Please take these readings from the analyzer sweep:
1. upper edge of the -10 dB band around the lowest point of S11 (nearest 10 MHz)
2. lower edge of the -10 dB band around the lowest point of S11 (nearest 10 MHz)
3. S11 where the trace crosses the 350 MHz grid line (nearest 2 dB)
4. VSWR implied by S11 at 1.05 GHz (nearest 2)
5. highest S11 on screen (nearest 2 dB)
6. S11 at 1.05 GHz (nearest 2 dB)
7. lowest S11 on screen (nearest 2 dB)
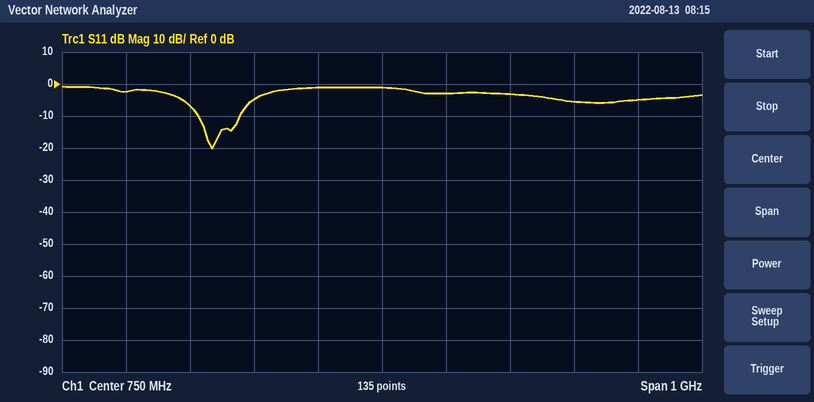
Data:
530 MHz
460 MHz
-2 dB
4
0 dB
-6 dB
-20 dB
